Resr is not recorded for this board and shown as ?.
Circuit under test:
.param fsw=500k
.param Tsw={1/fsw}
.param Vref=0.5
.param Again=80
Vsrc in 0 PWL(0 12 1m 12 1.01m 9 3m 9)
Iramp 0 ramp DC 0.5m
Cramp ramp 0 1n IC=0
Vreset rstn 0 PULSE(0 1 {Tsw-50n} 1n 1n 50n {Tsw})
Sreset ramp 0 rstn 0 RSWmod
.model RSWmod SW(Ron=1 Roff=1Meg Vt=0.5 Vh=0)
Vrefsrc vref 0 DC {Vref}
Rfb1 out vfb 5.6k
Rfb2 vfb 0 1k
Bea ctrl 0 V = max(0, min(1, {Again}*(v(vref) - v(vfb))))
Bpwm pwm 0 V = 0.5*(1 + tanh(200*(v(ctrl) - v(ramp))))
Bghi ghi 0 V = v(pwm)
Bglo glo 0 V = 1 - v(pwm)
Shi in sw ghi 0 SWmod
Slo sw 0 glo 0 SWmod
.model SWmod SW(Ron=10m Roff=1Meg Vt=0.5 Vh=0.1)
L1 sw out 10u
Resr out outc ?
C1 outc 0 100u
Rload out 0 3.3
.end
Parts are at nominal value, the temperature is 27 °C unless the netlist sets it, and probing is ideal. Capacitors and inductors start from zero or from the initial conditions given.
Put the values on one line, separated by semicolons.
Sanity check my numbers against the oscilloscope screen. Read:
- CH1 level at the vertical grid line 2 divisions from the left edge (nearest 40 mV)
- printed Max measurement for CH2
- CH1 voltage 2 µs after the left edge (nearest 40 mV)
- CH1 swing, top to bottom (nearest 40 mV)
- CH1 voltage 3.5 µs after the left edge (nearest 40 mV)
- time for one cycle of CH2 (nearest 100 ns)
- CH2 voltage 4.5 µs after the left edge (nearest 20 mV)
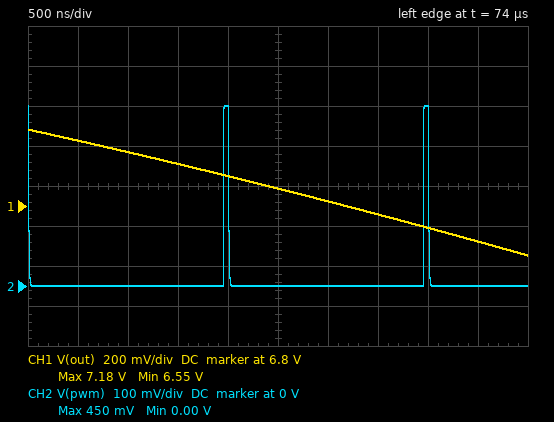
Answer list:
7.08 V; 450 mV; 6.96 V; 640 mV; 6.76 V; 2.0 µs; 0 V
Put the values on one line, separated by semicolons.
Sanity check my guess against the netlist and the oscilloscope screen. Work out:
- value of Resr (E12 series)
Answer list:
3.3 mΩ
